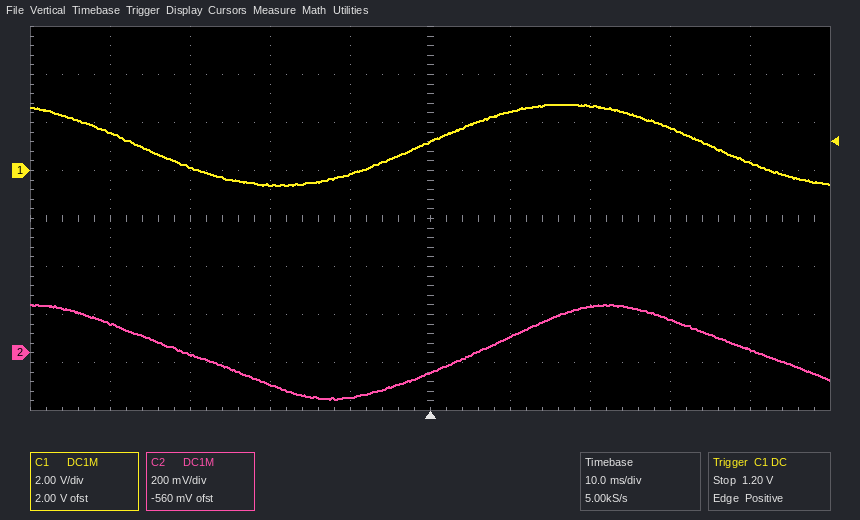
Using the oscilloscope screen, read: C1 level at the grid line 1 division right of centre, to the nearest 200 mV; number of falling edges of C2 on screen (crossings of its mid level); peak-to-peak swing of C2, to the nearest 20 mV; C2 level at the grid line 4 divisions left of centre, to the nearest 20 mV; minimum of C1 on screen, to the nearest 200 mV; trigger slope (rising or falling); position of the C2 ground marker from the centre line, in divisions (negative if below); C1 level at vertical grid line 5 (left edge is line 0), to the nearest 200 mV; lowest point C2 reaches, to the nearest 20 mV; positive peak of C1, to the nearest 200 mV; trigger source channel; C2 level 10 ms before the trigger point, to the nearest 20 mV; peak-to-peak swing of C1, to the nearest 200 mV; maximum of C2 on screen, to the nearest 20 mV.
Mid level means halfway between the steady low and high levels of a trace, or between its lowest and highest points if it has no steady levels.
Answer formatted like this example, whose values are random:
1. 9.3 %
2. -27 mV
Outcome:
1. 2.4 V
2. 2
3. 400 mV
4. 120 mV
5. -600 mV
6. rising
7. -2.8 div
8. 1.2 V
9. -200 mV
10. 2.8 V
11. C1
12. -180 mV
13. 3.4 V
14. 200 mV
